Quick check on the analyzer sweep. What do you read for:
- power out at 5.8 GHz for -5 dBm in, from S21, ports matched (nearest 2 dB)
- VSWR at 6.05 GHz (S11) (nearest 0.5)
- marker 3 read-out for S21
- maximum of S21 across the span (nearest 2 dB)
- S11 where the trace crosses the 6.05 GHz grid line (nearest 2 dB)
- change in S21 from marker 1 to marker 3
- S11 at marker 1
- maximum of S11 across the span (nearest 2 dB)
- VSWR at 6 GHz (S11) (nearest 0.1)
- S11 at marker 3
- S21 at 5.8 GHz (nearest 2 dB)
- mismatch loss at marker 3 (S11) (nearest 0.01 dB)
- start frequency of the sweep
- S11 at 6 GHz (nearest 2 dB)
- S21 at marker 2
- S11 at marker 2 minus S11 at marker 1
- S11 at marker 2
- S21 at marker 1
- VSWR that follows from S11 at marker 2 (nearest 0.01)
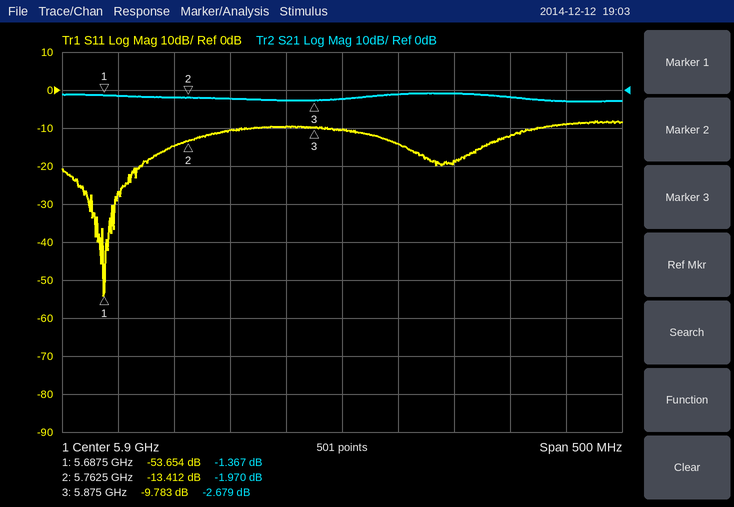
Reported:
-8 dBm
1.5
-2.679 dB
0 dB
-12 dB
-1.312 dB
-53.654 dB
-8 dB
1.3
-9.783 dB
-2 dB
0.48 dB
5.65 GHz
-18 dB
-1.970 dB
40.242 dB
-13.412 dB
-1.367 dB
1.54
